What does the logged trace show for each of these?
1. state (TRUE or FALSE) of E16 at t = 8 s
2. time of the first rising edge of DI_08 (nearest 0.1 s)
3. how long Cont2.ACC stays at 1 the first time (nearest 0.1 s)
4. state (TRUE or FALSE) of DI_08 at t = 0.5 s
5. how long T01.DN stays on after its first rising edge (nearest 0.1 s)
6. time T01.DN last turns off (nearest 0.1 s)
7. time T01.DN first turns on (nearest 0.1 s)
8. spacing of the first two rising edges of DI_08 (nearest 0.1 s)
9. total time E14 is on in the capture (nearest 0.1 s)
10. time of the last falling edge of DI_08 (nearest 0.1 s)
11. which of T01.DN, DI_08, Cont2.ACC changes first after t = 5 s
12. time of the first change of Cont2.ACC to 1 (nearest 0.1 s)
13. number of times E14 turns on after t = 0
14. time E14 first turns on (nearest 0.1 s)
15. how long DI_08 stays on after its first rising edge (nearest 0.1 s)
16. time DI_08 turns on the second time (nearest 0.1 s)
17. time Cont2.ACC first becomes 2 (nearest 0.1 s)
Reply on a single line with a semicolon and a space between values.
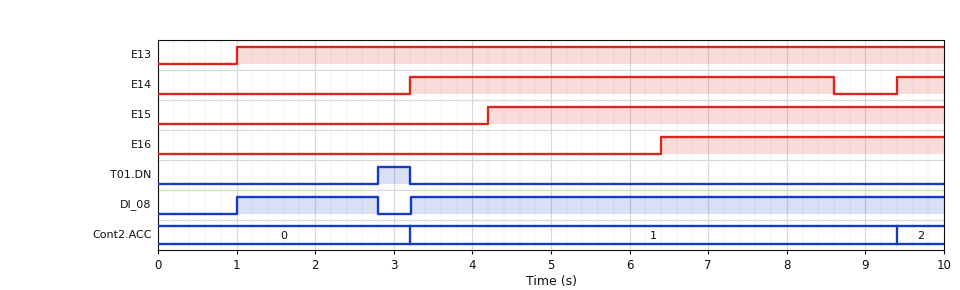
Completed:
TRUE; 1.0 s; 6.2 s; FALSE; 0.4 s; 3.2 s; 2.8 s; 2.2 s; 6.0 s; 2.8 s; Cont2.ACC; 3.2 s; 2; 3.2 s; 1.8 s; 3.2 s; 9.4 s
